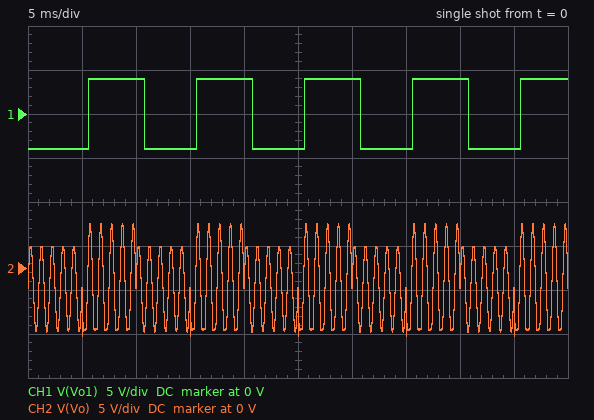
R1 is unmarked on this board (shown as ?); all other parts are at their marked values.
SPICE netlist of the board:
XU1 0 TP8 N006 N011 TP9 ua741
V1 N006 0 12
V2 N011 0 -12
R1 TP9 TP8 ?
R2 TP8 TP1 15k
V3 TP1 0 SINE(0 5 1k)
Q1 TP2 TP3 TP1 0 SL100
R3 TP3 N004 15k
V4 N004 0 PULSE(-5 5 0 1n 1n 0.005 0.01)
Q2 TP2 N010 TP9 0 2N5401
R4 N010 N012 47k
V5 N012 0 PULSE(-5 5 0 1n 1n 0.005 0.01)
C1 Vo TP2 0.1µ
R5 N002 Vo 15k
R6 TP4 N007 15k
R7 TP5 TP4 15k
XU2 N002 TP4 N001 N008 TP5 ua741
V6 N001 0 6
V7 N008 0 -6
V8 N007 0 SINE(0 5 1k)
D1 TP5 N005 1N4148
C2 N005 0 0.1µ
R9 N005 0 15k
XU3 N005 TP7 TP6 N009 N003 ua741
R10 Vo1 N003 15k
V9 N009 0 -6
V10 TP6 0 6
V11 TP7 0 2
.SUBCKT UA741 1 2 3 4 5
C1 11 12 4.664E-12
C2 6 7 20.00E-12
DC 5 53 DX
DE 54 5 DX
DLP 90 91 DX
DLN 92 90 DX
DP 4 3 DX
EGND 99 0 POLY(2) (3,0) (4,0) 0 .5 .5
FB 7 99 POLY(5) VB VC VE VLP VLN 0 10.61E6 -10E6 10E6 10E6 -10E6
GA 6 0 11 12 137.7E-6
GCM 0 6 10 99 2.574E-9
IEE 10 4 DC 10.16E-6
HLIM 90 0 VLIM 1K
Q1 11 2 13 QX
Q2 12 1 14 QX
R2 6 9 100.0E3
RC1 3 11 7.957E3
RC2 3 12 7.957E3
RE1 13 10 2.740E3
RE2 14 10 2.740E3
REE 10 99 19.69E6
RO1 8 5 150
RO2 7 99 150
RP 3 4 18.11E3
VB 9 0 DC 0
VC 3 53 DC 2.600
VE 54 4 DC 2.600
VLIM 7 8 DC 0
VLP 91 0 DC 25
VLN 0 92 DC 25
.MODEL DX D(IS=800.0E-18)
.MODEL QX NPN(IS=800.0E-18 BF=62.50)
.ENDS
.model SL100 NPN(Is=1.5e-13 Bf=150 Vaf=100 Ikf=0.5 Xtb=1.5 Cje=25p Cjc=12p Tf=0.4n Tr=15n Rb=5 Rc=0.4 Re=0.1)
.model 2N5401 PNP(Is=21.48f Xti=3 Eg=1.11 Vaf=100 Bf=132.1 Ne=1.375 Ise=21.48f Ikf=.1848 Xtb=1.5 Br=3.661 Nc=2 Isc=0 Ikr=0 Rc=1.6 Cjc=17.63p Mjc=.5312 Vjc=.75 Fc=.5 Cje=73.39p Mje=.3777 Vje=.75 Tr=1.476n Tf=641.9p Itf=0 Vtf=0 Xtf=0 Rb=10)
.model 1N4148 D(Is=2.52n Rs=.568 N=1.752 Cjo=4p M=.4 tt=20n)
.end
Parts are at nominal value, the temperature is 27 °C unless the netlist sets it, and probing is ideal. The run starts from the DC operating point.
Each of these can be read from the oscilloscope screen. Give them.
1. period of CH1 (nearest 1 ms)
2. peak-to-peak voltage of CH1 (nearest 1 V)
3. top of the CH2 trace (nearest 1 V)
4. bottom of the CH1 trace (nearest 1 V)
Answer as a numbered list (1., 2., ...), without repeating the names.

1. 10 ms
2. 8 V
3. 5 V
4. -4 V
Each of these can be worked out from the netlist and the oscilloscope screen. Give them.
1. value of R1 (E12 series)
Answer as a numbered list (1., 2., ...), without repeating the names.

1. 22 kΩ
